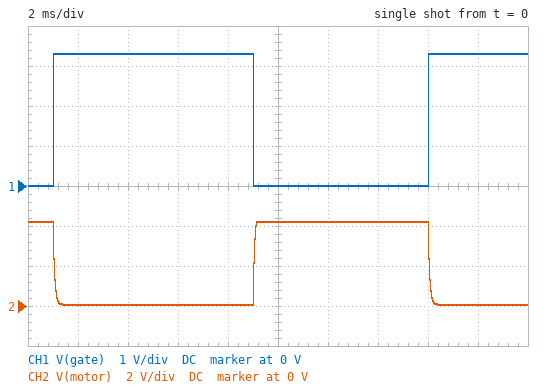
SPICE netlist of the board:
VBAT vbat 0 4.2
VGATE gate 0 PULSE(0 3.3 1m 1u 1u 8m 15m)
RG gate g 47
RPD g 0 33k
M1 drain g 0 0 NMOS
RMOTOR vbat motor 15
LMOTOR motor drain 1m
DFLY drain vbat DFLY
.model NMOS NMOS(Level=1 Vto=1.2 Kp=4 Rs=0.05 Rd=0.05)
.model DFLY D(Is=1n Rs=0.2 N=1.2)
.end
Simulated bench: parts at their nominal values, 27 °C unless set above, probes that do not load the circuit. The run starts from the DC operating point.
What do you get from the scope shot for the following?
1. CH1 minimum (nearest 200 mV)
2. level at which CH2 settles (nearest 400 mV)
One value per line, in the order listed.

0 V
0 V
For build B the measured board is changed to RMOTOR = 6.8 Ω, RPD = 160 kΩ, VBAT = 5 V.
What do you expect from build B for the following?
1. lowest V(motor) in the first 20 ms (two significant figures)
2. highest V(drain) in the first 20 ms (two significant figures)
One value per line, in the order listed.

160 mV
5.8 V
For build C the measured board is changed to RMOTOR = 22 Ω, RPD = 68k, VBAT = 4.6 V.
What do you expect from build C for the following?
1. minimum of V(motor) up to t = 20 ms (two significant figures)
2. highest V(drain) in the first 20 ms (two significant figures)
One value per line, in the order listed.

46 mV
5.2 V
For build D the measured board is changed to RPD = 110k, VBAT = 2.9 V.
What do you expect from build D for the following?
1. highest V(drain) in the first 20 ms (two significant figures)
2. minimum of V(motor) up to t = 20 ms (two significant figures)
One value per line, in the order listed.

3.5 V
42 mV
